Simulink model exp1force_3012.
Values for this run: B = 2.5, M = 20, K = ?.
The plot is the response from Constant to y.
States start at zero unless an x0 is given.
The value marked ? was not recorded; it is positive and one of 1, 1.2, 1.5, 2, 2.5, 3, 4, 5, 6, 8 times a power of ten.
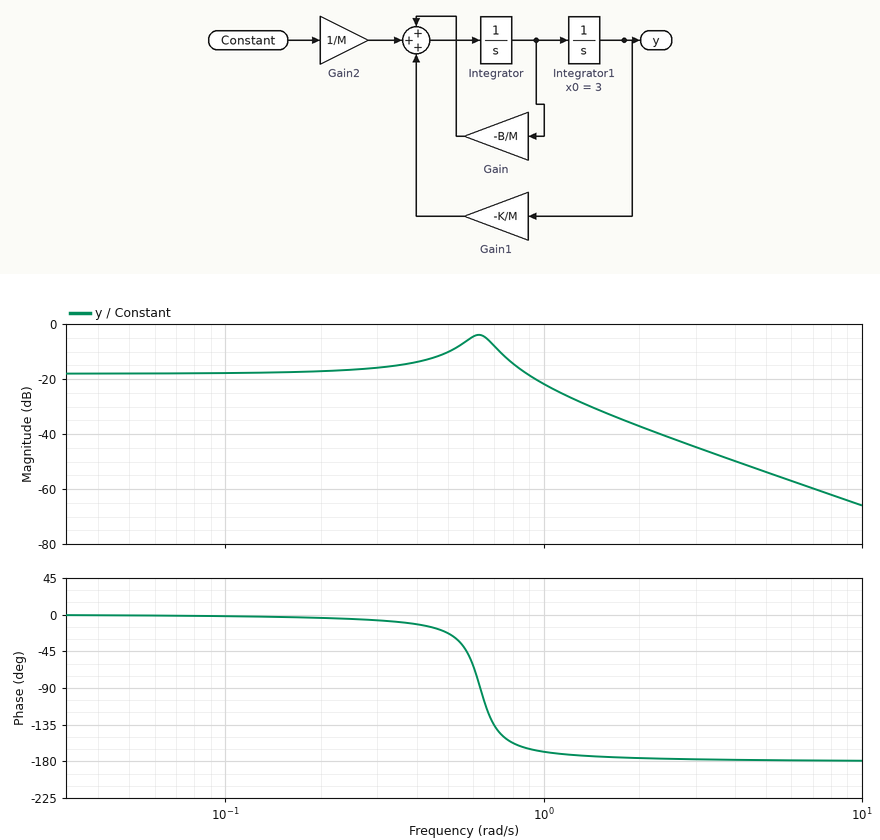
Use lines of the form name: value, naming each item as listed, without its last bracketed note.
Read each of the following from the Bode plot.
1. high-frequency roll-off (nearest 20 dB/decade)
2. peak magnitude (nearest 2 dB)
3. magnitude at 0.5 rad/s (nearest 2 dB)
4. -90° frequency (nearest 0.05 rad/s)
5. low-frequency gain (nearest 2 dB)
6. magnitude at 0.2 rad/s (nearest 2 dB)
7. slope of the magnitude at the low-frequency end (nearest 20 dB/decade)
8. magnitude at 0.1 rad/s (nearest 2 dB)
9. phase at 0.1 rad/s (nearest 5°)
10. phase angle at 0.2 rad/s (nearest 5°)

high-frequency roll-off: -40 dB/decade
peak magnitude: -4 dB
magnitude at 0.5 rad/s: -10 dB
-90° frequency: 0.65 rad/s
low-frequency gain: -18 dB
magnitude at 0.2 rad/s: -18 dB
slope of the magnitude at the low-frequency end: 0 dB/decade
magnitude at 0.1 rad/s: -18 dB
phase at 0.1 rad/s: 0°
phase angle at 0.2 rad/s: -5°
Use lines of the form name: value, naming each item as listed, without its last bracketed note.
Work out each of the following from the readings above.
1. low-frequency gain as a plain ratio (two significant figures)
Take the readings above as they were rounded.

low-frequency gain as a plain ratio: 0.13
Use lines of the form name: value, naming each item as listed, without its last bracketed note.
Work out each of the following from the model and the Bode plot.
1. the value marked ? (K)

the value marked ?: 8
